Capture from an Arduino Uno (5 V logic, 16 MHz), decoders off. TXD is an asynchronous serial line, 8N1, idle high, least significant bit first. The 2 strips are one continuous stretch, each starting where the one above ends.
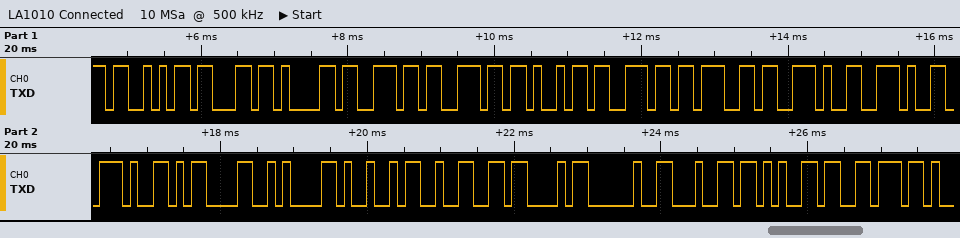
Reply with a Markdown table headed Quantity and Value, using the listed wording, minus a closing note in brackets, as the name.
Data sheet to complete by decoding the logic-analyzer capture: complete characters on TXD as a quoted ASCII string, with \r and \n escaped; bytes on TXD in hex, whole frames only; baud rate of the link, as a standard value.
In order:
| Quantity | Value |
|---|---|
| complete characters on TXD as a quoted ASCII string, with \r and \n escaped | "Scanning...\r\nI2C dev" |
| bytes on TXD in hex, whole frames only | 0x53 0x63 0x61 0x6E 0x6E 0x69 0x6E 0x67 0x2E 0x2E 0x2E 0x0D 0x0A 0x49 0x32 0x43 0x20 0x64 0x65 0x76 |
| baud rate of the link, as a standard value | 9600 baud |
